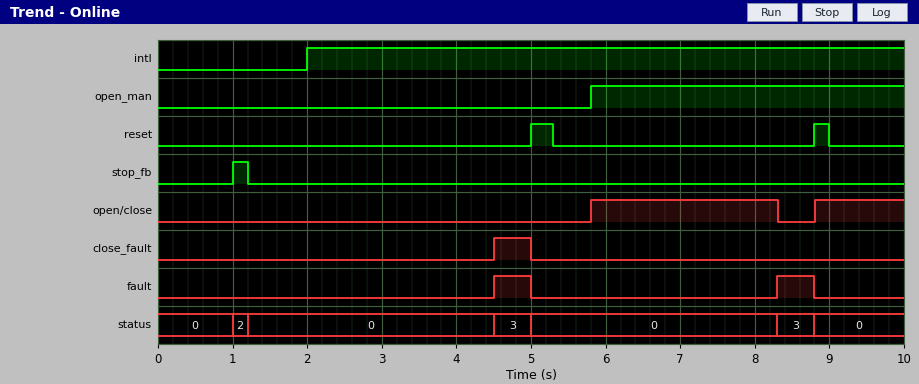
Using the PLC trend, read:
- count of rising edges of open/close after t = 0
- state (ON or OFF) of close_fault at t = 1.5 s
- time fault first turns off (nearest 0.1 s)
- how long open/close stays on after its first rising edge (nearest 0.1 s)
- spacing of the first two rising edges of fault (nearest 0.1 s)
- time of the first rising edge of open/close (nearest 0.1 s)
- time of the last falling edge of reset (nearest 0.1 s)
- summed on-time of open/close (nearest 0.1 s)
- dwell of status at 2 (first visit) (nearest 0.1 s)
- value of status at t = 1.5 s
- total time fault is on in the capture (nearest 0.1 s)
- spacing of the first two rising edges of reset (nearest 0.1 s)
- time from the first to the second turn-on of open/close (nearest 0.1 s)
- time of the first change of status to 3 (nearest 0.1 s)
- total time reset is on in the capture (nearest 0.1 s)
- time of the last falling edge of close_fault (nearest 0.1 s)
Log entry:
2
OFF
5.0 s
2.5 s
3.8 s
5.8 s
9.0 s
3.7 s
0.2 s
0
1.0 s
3.8 s
3.0 s
4.5 s
0.5 s
5.0 s
